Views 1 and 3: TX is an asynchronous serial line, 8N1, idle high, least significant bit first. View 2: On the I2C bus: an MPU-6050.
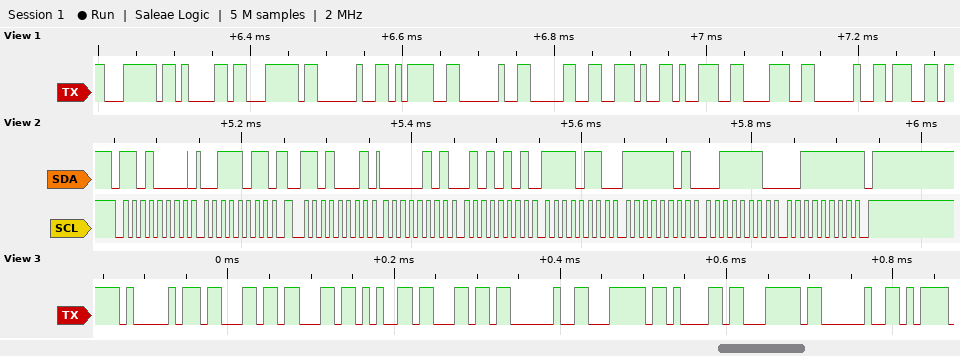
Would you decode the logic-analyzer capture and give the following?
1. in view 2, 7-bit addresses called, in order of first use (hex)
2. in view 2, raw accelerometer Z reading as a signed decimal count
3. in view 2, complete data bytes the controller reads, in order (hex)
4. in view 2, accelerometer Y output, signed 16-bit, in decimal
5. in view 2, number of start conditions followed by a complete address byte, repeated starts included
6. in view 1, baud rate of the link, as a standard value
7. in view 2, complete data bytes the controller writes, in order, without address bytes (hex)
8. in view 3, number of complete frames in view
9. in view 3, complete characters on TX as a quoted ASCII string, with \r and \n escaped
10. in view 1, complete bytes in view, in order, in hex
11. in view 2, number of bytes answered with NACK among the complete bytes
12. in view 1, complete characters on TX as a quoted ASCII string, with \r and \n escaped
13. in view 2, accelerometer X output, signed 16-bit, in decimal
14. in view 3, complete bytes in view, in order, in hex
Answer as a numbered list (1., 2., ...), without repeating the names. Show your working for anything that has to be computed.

1. 0x68
2. 0x3E3F = 15935
3. 05 55 F6 FD 3E 3F
4. 0xF6FD = -2307
5. 2
6. 115200 baud
7. 3B
8. 10
9. "Accel |a| "
10. 7C 61 7C 20 3D 20 30 2E 39 38 20 67
11. 1
12. "|a| = 0.98 g"
13. 0x0555 = 1365
14. 41 63 63 65 6C 20 7C 61 7C 20
